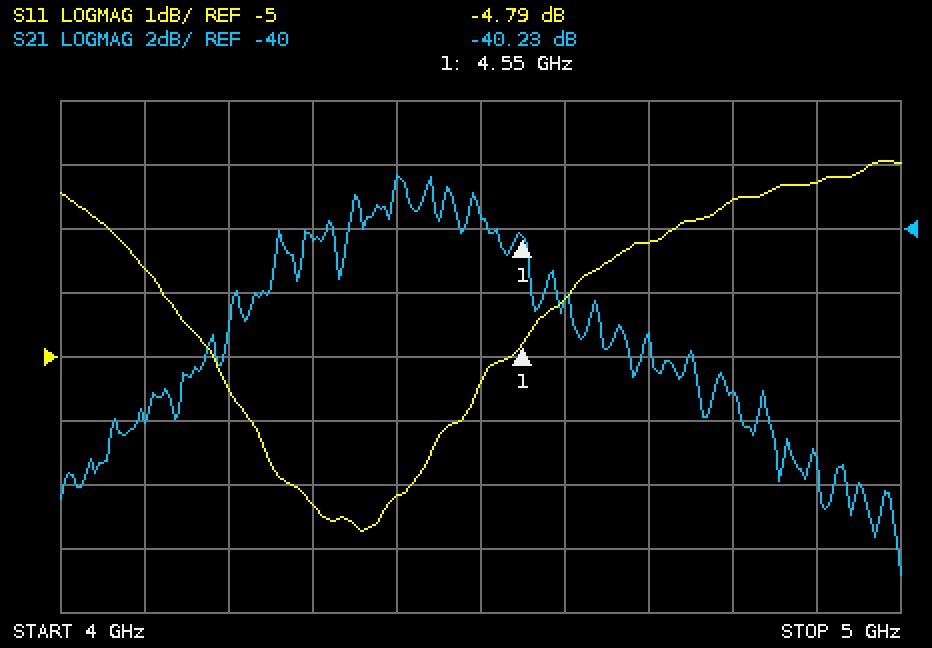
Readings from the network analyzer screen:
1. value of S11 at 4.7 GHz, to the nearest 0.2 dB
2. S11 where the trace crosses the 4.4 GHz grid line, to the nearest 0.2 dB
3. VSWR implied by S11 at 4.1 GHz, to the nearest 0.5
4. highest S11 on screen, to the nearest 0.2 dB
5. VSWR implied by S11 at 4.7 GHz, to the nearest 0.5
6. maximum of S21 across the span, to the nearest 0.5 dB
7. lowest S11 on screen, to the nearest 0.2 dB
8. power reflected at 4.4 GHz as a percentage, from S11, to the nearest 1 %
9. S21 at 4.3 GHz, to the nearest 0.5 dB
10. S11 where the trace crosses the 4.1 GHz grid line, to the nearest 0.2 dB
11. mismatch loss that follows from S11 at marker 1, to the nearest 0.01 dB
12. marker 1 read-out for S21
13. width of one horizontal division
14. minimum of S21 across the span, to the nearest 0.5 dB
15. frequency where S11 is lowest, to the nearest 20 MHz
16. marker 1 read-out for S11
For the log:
-3.2 dB
-7.2 dB
5.0
-2.0 dB
5.5
-38.5 dB
-7.8 dB
19 %
-40.5 dB
-3.6 dB
1.75 dB
-40.23 dB
100 MHz
-51.0 dB
4.36 GHz
-4.79 dB
